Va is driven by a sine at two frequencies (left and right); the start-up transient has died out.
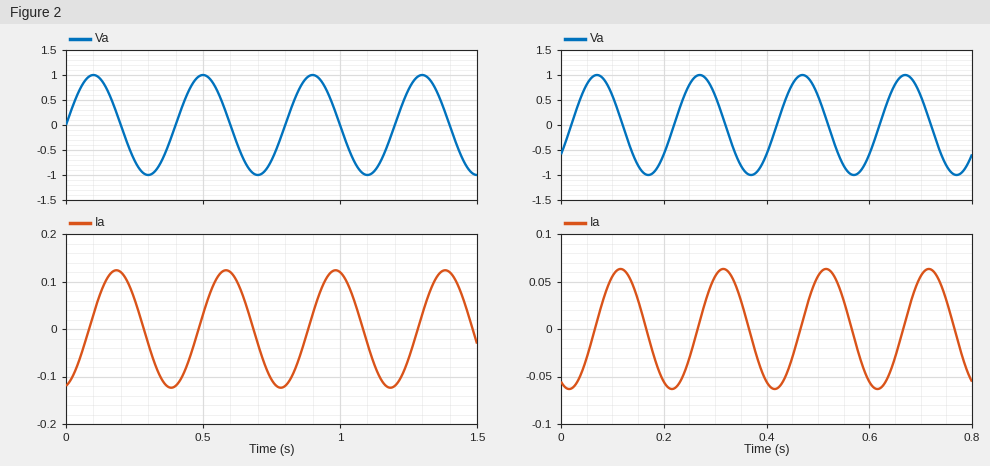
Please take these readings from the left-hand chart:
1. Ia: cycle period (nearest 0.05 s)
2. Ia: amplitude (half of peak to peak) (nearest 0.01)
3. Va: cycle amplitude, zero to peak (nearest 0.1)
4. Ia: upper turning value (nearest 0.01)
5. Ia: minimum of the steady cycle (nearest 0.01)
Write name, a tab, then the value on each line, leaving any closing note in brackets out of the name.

Ia: cycle period	0.40 s
Ia: amplitude (half of peak to peak)	0.12
Va: cycle amplitude, zero to peak	1.0
Ia: upper turning value	0.12
Ia: minimum of the steady cycle	-0.12
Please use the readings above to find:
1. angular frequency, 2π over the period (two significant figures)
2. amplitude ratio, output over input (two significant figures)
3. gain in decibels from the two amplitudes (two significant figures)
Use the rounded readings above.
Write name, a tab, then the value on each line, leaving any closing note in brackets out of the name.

angular frequency, 2π over the period	16 rad/s
amplitude ratio, output over input	0.12
gain in decibels from the two amplitudes	-18 dB
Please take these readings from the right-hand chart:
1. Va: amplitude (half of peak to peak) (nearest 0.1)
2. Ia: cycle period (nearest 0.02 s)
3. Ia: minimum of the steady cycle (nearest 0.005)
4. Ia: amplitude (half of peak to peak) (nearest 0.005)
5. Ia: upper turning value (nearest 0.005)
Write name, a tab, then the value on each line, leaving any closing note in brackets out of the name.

Va: amplitude (half of peak to peak)	1.0
Ia: cycle period	0.20 s
Ia: minimum of the steady cycle	-0.065
Ia: amplitude (half of peak to peak)	0.065
Ia: upper turning value	0.065
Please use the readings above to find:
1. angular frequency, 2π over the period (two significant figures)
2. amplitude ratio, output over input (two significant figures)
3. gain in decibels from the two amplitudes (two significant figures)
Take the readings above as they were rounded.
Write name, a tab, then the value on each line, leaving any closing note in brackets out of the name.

angular frequency, 2π over the period	31 rad/s
amplitude ratio, output over input	0.065
gain in decibels from the two amplitudes	-24 dB
